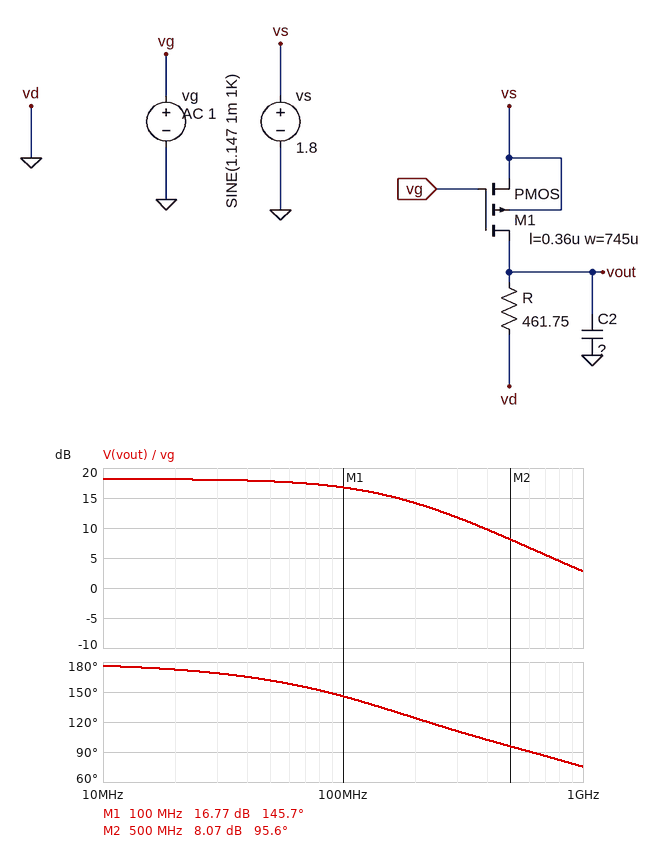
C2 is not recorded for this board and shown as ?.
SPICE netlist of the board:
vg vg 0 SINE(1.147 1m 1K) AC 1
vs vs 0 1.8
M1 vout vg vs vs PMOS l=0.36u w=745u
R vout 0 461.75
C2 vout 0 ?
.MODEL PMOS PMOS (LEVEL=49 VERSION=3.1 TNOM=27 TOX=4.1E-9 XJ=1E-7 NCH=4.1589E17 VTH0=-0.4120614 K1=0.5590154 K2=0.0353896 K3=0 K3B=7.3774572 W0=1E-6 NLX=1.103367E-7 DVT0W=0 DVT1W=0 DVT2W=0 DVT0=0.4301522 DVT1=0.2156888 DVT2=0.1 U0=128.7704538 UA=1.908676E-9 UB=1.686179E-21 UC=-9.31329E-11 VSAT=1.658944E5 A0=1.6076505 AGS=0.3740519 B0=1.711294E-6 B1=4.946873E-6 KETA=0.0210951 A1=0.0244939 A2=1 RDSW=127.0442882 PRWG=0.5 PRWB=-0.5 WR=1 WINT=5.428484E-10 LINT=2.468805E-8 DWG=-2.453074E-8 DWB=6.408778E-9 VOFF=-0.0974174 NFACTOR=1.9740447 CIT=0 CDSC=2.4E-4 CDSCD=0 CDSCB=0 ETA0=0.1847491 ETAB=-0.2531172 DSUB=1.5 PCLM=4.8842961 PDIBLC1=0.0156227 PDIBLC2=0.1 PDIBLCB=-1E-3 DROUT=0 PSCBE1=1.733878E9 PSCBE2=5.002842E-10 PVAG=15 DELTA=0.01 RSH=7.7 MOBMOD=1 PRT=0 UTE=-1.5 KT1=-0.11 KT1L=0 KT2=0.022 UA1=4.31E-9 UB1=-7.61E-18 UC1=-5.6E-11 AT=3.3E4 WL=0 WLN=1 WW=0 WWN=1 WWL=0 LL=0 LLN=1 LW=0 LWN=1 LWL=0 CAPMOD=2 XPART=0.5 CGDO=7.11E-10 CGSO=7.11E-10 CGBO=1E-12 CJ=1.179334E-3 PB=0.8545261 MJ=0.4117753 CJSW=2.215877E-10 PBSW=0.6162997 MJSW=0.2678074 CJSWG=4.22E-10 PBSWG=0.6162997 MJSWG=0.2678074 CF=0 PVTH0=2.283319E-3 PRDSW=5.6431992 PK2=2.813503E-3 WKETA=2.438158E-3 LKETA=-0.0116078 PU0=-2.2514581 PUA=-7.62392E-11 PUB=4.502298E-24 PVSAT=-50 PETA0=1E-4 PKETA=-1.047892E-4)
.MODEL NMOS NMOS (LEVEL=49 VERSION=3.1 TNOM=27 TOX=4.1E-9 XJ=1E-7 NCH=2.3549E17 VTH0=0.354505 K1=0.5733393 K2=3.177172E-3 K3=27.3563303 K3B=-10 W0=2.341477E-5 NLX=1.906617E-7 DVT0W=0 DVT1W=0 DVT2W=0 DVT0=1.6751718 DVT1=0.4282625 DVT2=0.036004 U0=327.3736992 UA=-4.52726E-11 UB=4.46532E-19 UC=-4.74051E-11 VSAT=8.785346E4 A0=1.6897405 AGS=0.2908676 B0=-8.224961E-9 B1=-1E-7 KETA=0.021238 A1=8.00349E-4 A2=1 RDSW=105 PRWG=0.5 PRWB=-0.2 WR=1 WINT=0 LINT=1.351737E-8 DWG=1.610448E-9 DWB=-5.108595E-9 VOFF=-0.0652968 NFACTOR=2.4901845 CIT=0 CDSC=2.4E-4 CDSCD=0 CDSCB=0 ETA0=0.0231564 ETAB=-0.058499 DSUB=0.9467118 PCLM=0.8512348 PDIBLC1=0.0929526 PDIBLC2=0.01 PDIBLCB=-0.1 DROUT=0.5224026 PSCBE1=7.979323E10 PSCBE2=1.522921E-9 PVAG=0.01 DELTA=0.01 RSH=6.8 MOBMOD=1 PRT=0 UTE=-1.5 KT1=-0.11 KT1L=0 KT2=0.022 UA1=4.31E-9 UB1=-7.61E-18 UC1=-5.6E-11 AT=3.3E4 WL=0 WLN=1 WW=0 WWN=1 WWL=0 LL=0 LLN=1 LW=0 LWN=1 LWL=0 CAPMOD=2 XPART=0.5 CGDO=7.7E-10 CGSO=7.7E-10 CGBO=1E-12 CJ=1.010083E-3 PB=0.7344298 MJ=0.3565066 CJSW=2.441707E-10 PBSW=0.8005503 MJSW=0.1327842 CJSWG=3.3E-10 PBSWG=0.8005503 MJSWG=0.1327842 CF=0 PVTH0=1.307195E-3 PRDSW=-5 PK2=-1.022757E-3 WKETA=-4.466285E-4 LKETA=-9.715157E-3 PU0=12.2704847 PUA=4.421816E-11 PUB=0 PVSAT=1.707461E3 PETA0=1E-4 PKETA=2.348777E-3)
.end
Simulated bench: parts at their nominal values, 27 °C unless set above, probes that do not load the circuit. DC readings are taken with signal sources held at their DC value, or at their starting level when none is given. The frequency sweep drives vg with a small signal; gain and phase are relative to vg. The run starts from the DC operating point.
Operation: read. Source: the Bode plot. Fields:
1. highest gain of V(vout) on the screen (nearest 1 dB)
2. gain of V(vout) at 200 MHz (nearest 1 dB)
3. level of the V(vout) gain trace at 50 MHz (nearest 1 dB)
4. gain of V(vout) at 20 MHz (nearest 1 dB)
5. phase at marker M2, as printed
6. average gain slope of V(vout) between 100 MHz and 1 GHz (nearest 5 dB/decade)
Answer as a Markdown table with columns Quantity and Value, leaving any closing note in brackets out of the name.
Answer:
| Quantity | Value |
|---|---|
| highest gain of V(vout) on the screen | 18 dB |
| gain of V(vout) at 200 MHz | 14 dB |
| level of the V(vout) gain trace at 50 MHz | 18 dB |
| gain of V(vout) at 20 MHz | 18 dB |
| phase at marker M2, as printed | 95.6 deg |
| average gain slope of V(vout) between 100 MHz and 1 GHz | -15 dB/decade |
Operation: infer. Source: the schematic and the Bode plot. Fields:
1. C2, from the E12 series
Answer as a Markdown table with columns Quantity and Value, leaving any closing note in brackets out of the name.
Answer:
| Quantity | Value |
|---|---|
| C2, from the E12 series | 1.5 pF |
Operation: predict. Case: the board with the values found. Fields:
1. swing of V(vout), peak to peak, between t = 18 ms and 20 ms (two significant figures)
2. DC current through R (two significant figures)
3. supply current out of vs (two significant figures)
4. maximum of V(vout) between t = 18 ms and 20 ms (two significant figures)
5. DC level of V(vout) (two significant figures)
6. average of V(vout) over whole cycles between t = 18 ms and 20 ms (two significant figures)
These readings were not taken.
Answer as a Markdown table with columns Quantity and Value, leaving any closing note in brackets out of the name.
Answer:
| Quantity | Value |
|---|---|
| swing of V(vout), peak to peak, between t = 18 ms and 20 ms | 16 mV |
| DC current through R | 2.1 mA |
| supply current out of vs | 2.1 mA |
| maximum of V(vout) between t = 18 ms and 20 ms | 960 mV |
| DC level of V(vout) | 950 mV |
| average of V(vout) over whole cycles between t = 18 ms and 20 ms | 950 mV |
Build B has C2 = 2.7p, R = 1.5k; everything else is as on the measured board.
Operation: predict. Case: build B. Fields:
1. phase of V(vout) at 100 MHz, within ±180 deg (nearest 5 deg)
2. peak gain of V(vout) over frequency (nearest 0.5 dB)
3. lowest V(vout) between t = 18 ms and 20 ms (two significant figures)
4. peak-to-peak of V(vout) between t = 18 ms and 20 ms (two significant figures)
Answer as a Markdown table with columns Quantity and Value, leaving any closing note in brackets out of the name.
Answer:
| Quantity | Value |
|---|---|
| phase of V(vout) at 100 MHz, within ±180 deg | 160 deg |
| peak gain of V(vout) over frequency | -6.0 dB |
| lowest V(vout) between t = 18 ms and 20 ms | 1.7 V |
| peak-to-peak of V(vout) between t = 18 ms and 20 ms | 1.0 mV |
